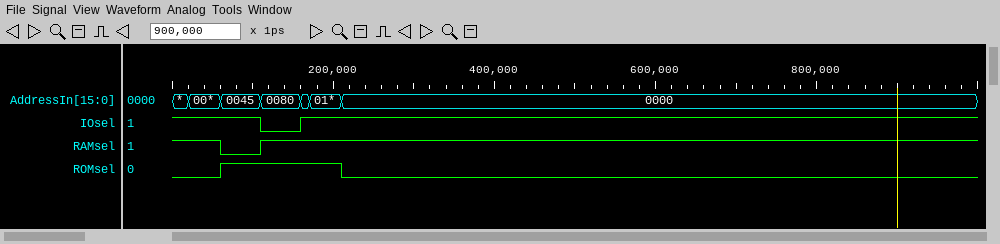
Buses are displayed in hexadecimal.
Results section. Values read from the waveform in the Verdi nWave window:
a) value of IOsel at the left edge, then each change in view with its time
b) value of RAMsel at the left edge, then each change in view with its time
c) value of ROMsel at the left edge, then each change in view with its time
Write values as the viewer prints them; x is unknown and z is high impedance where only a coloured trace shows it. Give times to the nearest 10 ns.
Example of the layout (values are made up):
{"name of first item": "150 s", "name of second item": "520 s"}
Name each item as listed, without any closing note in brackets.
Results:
{"value of IOsel at the left edge, then each change in view with its time": "1, 0 at 110 ns, 1 at 160 ns", "value of RAMsel at the left edge, then each change in view with its time": "1, 0 at 60 ns, 1 at 110 ns", "value of ROMsel at the left edge, then each change in view with its time": "0, 1 at 60 ns, 0 at 210 ns"}
